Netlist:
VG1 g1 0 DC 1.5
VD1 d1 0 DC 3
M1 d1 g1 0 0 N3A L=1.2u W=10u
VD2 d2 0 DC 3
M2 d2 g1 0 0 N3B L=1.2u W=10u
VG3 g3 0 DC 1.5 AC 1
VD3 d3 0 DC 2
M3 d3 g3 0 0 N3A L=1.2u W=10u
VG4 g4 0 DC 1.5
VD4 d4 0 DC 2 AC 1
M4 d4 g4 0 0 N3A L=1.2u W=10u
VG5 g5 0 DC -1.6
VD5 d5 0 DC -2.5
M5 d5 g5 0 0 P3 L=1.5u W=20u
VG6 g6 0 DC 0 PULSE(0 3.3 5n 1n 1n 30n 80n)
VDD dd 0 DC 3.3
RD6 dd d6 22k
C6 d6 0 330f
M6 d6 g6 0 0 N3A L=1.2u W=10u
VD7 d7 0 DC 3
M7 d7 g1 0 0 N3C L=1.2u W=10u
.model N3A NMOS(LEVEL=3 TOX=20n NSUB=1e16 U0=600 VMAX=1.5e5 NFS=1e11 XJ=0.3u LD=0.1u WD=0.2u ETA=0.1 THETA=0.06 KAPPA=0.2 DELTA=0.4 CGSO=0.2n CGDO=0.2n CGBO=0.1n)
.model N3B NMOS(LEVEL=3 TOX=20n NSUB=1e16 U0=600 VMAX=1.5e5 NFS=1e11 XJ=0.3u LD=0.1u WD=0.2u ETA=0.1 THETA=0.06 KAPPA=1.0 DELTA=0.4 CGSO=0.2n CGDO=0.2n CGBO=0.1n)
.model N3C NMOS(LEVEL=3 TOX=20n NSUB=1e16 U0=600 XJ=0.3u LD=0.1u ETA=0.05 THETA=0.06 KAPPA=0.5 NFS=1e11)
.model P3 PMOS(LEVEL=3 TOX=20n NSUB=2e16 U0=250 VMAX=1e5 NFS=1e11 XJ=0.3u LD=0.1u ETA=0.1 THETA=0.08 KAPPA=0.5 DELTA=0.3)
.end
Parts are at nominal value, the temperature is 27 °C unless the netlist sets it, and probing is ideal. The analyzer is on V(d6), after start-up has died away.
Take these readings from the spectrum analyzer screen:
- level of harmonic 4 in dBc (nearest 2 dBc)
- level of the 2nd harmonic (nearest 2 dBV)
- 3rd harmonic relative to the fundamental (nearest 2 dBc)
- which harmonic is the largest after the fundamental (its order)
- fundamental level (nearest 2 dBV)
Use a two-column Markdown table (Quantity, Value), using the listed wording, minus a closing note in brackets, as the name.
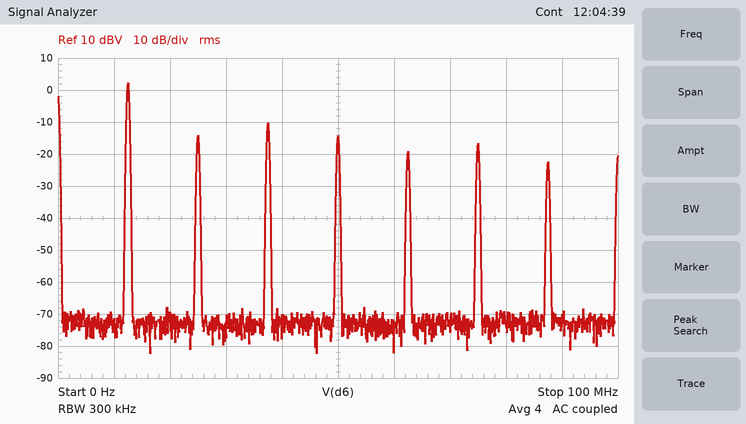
| Quantity | Value |
|---|---|
| level of harmonic 4 in dBc | -16 dBc |
| level of the 2nd harmonic | -14 dBV |
| 3rd harmonic relative to the fundamental | -12 dBc |
| which harmonic is the largest after the fundamental | 3 |
| fundamental level | 2 dBV |
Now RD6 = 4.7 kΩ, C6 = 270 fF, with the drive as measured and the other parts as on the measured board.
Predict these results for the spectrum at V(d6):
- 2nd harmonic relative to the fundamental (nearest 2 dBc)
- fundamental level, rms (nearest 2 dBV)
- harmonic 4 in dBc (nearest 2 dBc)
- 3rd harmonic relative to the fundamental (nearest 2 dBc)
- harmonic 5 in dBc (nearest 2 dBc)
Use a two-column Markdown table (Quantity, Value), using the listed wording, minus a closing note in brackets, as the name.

| Quantity | Value |
|---|---|
| 2nd harmonic relative to the fundamental | -10 dBc |
| fundamental level, rms | 2 dBV |
| harmonic 4 in dBc | -12 dBc |
| 3rd harmonic relative to the fundamental | -14 dBc |
| harmonic 5 in dBc | -40 dBc |
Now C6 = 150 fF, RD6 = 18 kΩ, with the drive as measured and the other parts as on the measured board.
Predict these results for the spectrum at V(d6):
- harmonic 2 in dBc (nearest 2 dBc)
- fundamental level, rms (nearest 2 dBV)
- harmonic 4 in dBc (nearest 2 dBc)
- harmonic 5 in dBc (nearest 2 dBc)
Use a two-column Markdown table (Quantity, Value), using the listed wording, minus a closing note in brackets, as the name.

| Quantity | Value |
|---|---|
| harmonic 2 in dBc | -12 dBc |
| fundamental level, rms | 2 dBV |
| harmonic 4 in dBc | -14 dBc |
| harmonic 5 in dBc | -26 dBc |
